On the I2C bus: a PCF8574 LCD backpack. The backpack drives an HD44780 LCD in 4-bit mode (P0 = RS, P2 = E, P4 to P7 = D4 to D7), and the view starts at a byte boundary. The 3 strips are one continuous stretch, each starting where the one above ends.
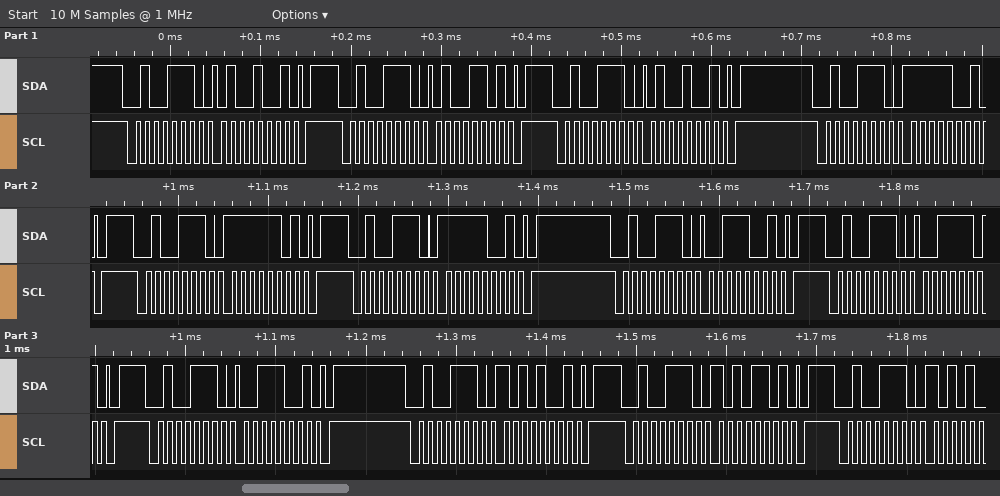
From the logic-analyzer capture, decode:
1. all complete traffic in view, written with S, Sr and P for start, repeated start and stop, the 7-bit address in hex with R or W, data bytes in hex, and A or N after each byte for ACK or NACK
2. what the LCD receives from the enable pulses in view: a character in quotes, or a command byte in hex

S 27W A 49 A P S 27W A 4D A P S 27W A 49 A P S 27W A F9 A P S 27W A FD A P S 27W A F9 A P S 27W A 39 A P S 27W A 3D A P S 27W A 39 A P S 27W A A9 A P S 27W A AD A P S 27W A
'O'
